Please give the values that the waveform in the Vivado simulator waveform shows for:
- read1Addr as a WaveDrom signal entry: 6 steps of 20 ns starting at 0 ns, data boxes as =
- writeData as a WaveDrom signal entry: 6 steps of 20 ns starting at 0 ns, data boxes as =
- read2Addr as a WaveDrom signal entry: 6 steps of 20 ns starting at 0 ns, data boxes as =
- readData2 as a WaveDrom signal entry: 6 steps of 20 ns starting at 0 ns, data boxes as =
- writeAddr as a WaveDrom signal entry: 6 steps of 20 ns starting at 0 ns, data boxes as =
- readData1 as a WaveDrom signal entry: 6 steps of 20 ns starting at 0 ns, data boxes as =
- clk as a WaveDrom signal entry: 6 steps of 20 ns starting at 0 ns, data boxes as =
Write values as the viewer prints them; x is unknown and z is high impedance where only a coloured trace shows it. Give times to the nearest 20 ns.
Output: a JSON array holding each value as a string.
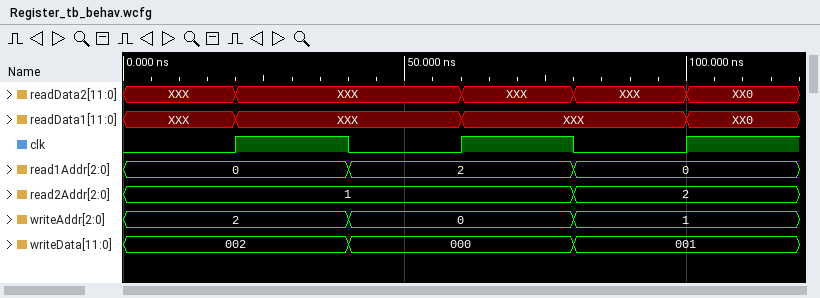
["{name: 'read1Addr', wave: '=.=.=.', data: '0 2 0'}", "{name: 'writeData', wave: '=.=.=.', data: '002 000 001'}", "{name: 'read2Addr', wave: '=...=.', data: '1 2'}", "{name: 'readData2', wave: 'x=.===', data: 'XXX XXX XXX XX0'}", "{name: 'writeAddr', wave: '=.=.=.', data: '2 0 1'}", "{name: 'readData1', wave: 'x=.=.=', data: 'XXX XXX XX0'}", "{name: 'clk', wave: '010101'}"]
